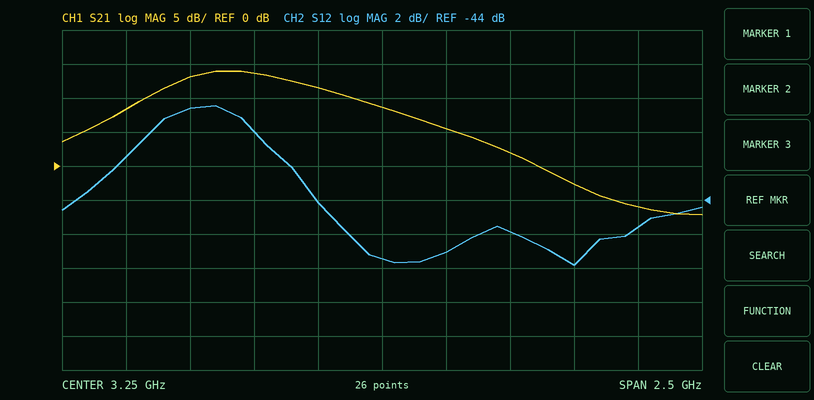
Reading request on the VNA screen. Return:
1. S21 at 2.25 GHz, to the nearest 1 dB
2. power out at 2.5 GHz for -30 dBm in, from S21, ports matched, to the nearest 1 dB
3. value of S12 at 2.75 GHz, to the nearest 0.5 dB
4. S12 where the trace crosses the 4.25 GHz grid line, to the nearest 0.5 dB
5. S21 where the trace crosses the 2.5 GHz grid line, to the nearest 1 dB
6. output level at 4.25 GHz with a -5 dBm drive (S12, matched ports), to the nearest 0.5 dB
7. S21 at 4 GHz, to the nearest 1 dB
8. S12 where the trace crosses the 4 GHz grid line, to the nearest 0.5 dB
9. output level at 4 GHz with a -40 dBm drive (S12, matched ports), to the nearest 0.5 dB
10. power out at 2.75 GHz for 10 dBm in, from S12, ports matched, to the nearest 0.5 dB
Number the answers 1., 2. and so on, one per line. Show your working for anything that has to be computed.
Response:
1. 8 dB
2. -30 dBm + (13 dB) = -17 dBm
3. -40.0 dB
4. -45.5 dB
5. 13 dB
6. -5 dBm + (-45.5 dB) = -50.5 dBm
7. -3 dB
8. -48.0 dB
9. -40 dBm + (-48.0 dB) = -88.0 dBm
10. 10 dBm + (-40.0 dB) = -30.0 dBm
